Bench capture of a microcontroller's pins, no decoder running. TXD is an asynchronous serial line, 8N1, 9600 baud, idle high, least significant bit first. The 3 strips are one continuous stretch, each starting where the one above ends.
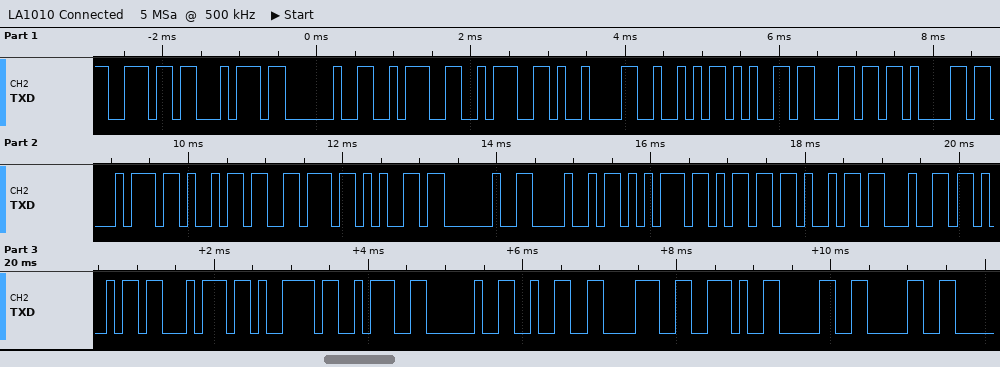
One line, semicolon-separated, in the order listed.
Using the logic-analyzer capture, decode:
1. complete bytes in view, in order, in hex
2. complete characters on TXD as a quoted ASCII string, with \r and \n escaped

6E 74 20 3A 3A 09 52 65 6C 61 74 69 76 65 20 48 75 6D 69 64 69 74 79 3A 20 32 38 2E 30 30; "nt ::\tRelative Humidity: 28.00"
